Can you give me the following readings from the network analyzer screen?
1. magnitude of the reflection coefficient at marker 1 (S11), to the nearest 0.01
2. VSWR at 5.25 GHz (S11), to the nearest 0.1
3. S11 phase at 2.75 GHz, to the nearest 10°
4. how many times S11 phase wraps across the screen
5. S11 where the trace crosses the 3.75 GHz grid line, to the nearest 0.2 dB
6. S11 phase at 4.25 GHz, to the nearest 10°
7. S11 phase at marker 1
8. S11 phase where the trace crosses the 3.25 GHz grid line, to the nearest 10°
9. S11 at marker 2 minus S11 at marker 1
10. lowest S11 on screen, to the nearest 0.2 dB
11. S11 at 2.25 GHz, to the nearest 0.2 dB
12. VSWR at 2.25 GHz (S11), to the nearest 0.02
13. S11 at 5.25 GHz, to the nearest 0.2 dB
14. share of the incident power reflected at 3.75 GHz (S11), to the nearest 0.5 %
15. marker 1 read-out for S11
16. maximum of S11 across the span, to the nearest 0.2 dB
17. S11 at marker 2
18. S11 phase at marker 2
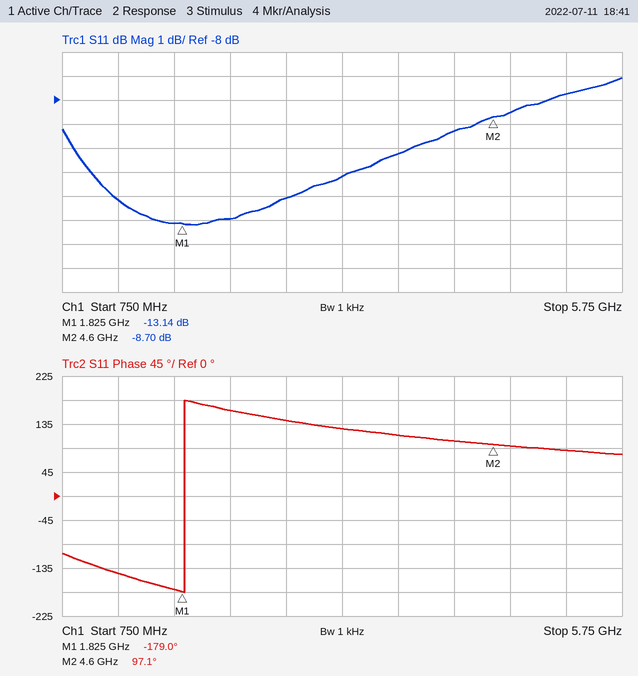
0.22
2.4
140°
1
-10.2 dB
100°
-179.0°
130°
4.44 dB
-13.2 dB
-13.0 dB
1.58
-7.8 dB
9.5 %
-13.14 dB
-7.0 dB
-8.70 dB
97.1°
